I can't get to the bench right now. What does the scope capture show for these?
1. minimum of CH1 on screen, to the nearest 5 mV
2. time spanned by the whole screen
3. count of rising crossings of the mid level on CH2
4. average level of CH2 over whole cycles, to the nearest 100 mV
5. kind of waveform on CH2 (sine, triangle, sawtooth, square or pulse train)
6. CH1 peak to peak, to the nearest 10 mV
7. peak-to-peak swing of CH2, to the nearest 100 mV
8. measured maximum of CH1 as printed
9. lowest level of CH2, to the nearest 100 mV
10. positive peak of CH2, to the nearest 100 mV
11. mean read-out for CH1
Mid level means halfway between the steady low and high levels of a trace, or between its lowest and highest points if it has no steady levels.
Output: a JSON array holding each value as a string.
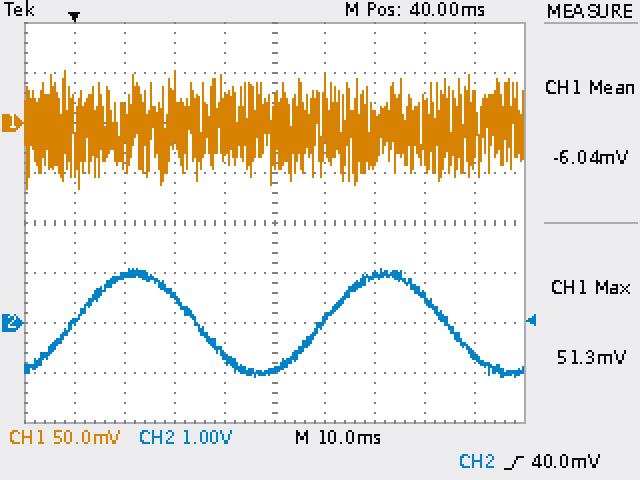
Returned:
["-65 mV", "100 ms", "2", "0.0 V", "sine", "120 mV", "2.2 V", "51.3 mV", "-1.1 V", "1.1 V", "-6.04 mV"]
